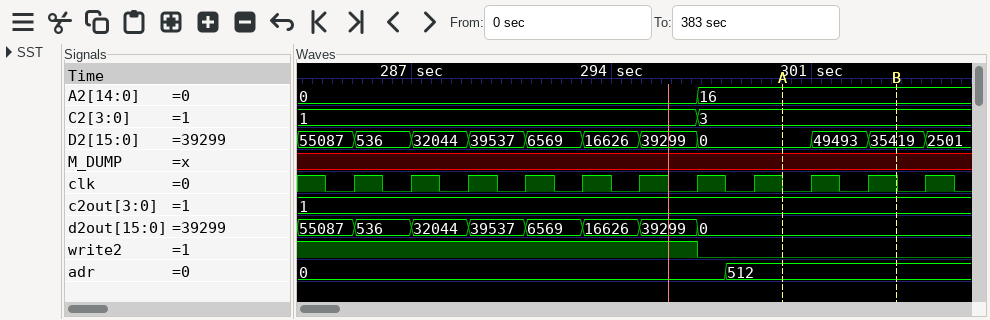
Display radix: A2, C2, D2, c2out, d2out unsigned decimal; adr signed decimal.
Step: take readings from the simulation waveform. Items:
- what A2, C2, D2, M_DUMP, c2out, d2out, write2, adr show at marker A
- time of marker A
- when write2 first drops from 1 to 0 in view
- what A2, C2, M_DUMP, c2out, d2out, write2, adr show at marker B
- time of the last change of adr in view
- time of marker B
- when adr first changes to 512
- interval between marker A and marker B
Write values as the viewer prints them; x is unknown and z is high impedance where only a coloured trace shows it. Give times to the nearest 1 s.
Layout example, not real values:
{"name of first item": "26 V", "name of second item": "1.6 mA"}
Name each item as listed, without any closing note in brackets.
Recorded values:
{"what A2, C2, D2, M_DUMP, c2out, d2out, write2, adr show at marker A": "A2=16, C2=3, D2=0, M_DUMP=x, c2out=1, d2out=0, write2=0, adr=512", "time of marker A": "300 s", "when write2 first drops from 1 to 0 in view": "297 s", "what A2, C2, M_DUMP, c2out, d2out, write2, adr show at marker B": "A2=16, C2=3, M_DUMP=x, c2out=1, d2out=0, write2=0, adr=512", "time of the last change of adr in view": "298 s", "time of marker B": "304 s", "when adr first changes to 512": "298 s", "interval between marker A and marker B": "4 s"}
